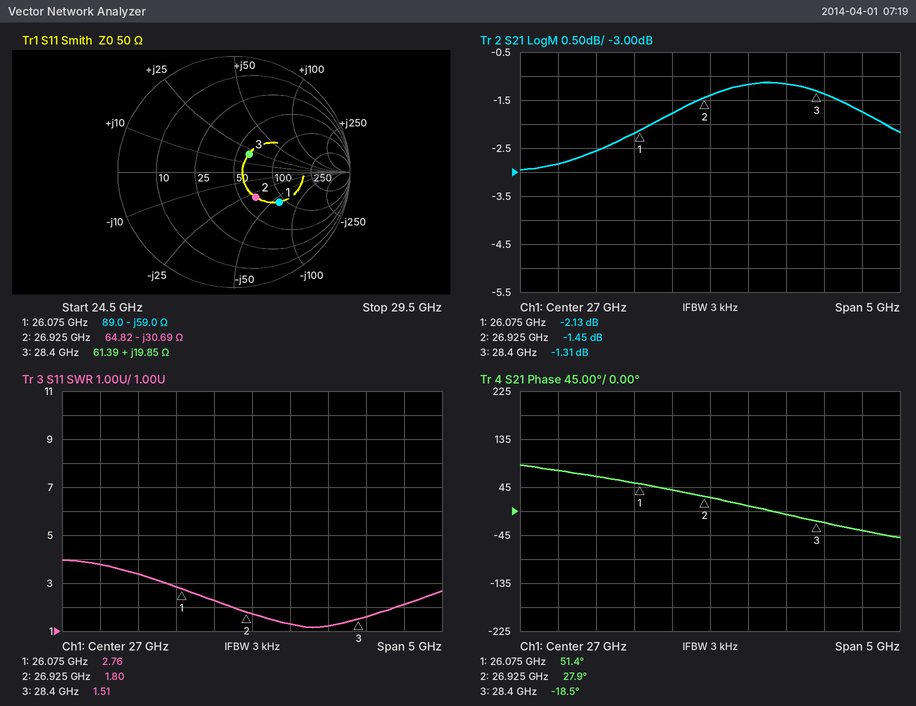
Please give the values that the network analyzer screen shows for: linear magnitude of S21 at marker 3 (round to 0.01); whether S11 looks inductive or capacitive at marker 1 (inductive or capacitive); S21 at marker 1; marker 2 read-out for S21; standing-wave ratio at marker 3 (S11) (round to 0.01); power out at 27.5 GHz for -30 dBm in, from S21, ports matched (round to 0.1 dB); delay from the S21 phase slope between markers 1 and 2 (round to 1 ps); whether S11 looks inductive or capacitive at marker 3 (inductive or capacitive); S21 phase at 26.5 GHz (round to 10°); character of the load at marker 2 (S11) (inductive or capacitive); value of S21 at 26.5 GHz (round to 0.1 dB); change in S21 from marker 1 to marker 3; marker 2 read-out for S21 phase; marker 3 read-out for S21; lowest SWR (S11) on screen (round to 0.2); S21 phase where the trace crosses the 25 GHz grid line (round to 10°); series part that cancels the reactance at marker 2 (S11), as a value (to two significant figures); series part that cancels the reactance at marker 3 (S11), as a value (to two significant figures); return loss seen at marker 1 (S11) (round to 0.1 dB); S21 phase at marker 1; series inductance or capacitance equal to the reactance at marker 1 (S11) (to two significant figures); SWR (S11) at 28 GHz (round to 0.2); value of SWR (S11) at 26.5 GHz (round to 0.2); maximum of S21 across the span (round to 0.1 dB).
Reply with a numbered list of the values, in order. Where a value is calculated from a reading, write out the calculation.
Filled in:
1. 10^(-1.31/20) ≈ 0.86
2. capacitive
3. -2.13 dB
4. -1.45 dB
5. 1.51
6. -30 dBm + (-1.2 dB) = -31.2 dBm
7. −(27.9° − (51.4°))/(360° × 850 MHz) ≈ 77 ps
8. inductive
9. 40°
10. capacitive
11. -1.8 dB
12. -1.31 − (-2.13) = 0.82 dB
13. 27.9°
14. -1.31 dB
15. 1.2
16. 80°
17. L = 30.69 Ω/(2π × 26.925 GHz) ≈ 181 pH, so 180 pH to two significant figures
18. C = 1/(2π × 28.4 GHz × 19.85 Ω) ≈ 282 fF, so 280 fF to two significant figures
19. 6.6 dB
20. 51.4°
21. C = 1/(2π × 26.075 GHz × 59 Ω) ≈ 103 fF, so 100 fF to two significant figures
22. 1.2
23. 2.2
24. -1.1 dB
